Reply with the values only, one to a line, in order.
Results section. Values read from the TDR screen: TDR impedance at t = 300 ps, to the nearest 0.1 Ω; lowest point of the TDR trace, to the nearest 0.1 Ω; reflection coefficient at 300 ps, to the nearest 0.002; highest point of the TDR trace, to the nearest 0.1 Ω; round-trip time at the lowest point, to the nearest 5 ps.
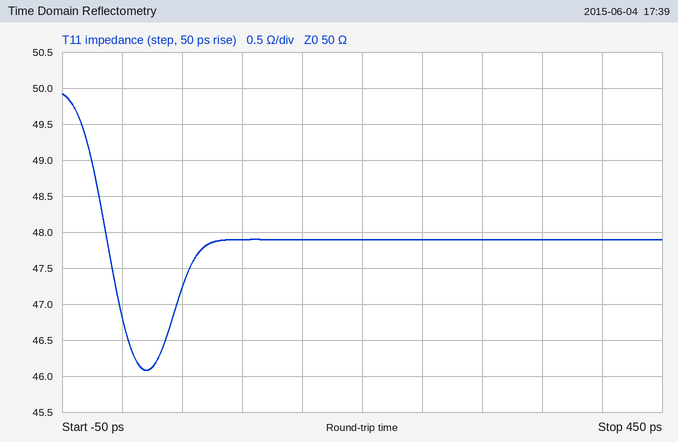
47.9 Ω
46.1 Ω
-0.022
49.9 Ω
20 ps
